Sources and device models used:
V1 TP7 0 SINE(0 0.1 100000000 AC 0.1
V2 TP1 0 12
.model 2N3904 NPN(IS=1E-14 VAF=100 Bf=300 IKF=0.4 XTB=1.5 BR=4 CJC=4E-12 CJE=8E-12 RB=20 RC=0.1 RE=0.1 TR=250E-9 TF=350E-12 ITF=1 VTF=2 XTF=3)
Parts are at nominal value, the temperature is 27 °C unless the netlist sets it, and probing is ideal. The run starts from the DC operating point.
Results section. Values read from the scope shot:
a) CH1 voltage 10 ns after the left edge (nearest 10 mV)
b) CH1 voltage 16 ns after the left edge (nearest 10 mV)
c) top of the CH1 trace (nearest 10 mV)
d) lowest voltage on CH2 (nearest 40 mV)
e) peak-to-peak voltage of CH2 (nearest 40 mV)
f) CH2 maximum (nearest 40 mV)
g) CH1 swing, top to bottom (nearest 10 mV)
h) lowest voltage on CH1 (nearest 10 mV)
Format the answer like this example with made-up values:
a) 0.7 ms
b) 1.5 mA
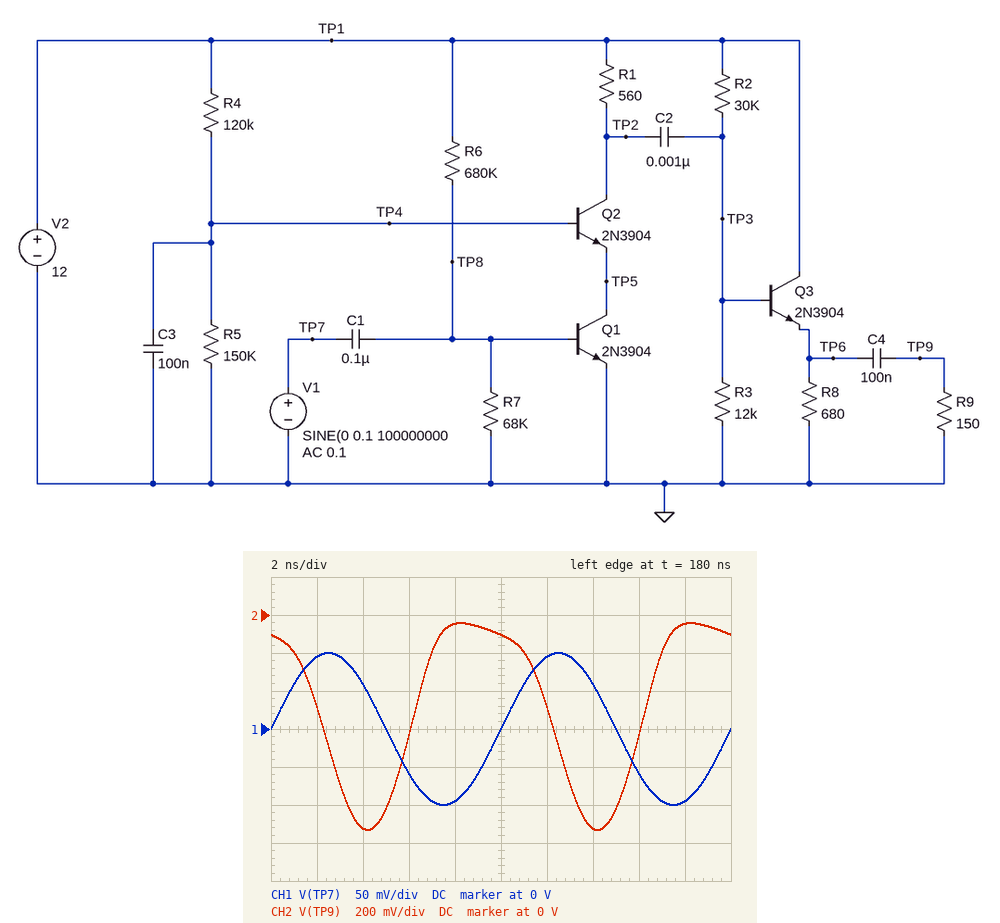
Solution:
a) 0 V
b) -60 mV
c) 100 mV
d) -1.12 V
e) 1.08 V
f) -40 mV
g) 200 mV
h) -100 mV
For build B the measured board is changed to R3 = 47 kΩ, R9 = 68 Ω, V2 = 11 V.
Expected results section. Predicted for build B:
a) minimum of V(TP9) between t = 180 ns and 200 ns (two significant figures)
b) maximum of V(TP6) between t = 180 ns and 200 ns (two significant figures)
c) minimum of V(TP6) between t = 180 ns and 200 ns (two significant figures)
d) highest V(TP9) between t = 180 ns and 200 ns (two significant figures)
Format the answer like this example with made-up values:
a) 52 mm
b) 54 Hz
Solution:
a) -820 mV
b) 5.2 V
c) 4.7 V
d) -300 mV
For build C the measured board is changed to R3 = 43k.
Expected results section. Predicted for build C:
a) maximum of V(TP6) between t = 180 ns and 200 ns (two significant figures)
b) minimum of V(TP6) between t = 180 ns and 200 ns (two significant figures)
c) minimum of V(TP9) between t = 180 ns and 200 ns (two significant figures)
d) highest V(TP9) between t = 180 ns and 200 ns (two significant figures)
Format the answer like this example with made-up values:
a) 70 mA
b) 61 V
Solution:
a) 5.2 V
b) 4.1 V
c) -1.7 V
d) -620 mV
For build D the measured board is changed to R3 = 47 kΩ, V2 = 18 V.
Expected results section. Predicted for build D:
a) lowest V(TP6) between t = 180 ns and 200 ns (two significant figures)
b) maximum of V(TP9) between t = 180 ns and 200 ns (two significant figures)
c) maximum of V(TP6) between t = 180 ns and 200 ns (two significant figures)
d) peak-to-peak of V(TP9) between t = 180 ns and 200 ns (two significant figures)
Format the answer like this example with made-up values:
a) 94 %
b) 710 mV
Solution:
a) 6.8 V
b) -1.0 V
c) 8.4 V
d) 1.6 V
